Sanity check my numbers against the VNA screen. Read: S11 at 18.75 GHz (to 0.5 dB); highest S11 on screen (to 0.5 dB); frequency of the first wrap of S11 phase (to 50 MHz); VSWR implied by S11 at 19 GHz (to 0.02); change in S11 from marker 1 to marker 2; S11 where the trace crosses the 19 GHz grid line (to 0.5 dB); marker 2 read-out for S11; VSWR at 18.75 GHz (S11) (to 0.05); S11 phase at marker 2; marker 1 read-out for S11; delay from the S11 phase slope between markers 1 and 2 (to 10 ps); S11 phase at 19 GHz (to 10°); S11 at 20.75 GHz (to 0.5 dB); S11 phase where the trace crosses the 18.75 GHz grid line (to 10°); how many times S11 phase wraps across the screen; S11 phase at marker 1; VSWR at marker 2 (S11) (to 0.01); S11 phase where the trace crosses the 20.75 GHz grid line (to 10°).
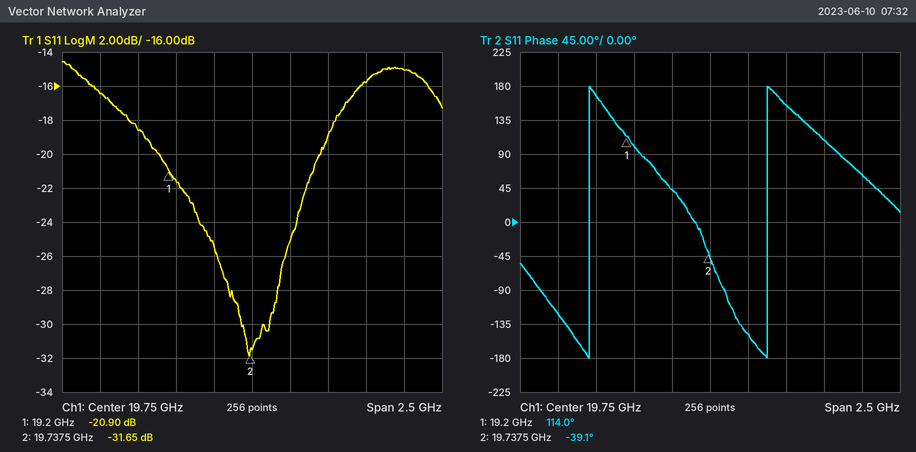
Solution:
-16.5 dB
-14.5 dB
18.95 GHz
1.26
-10.75 dB
-18.5 dB
-31.65 dB
1.35
-39.1°
-20.90 dB
790 ps
170°
-15.0 dB
-120°
2
114.0°
1.05
60°
